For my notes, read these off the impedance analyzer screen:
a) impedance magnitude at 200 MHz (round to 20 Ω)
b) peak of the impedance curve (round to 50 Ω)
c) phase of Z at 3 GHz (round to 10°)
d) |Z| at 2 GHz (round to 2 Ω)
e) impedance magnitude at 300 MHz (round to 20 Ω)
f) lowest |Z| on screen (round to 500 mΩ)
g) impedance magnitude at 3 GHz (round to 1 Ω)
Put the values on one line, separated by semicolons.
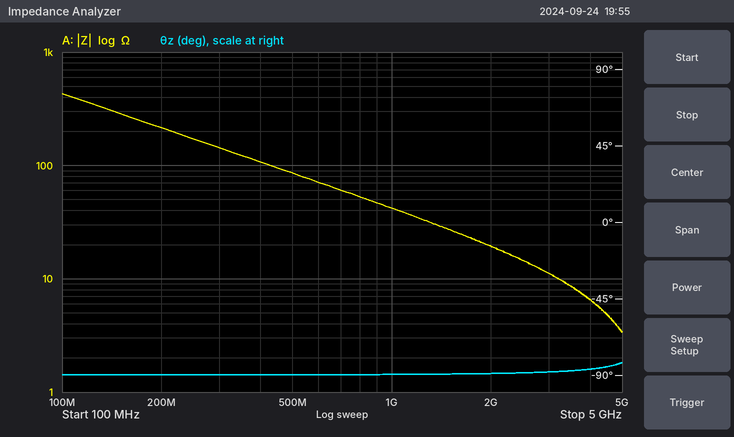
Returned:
220 Ω; 450 Ω; -90°; 20 Ω; 140 Ω; 3.5 Ω; 11 Ω
